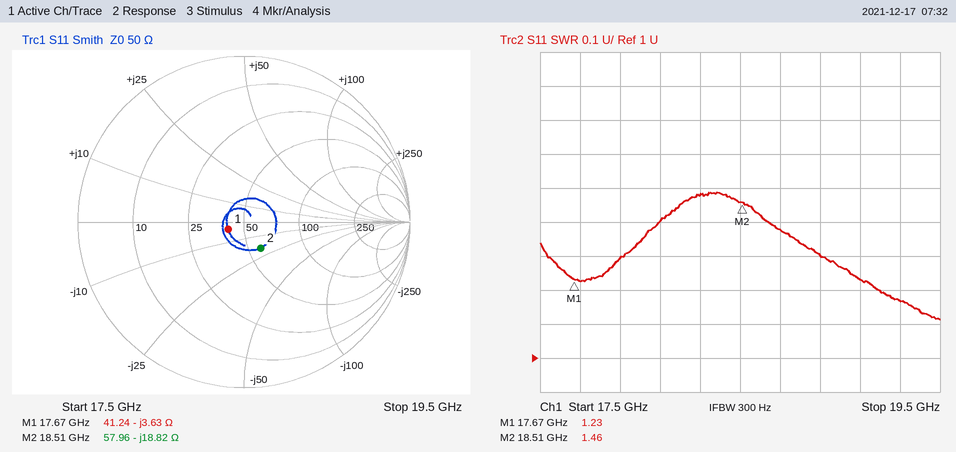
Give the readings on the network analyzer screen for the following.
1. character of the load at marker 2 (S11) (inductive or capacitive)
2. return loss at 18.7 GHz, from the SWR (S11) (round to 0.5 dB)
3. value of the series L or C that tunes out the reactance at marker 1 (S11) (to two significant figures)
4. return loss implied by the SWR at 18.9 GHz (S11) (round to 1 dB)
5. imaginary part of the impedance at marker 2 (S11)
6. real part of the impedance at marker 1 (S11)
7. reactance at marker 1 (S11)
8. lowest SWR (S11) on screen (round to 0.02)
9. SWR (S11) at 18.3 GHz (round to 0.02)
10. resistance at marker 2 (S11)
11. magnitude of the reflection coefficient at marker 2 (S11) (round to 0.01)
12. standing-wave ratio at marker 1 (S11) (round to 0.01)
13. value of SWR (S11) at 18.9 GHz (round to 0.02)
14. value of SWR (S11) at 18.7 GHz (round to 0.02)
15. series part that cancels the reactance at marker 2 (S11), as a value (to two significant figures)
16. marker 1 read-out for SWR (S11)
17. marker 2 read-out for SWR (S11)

capacitive
16.0 dB
33 pH
18 dB
-18.82 Ω
41.24 Ω
-3.63 Ω
1.12
1.48
57.96 Ω
0.19
1.23
1.30
1.38
160 pH
1.23
1.46
